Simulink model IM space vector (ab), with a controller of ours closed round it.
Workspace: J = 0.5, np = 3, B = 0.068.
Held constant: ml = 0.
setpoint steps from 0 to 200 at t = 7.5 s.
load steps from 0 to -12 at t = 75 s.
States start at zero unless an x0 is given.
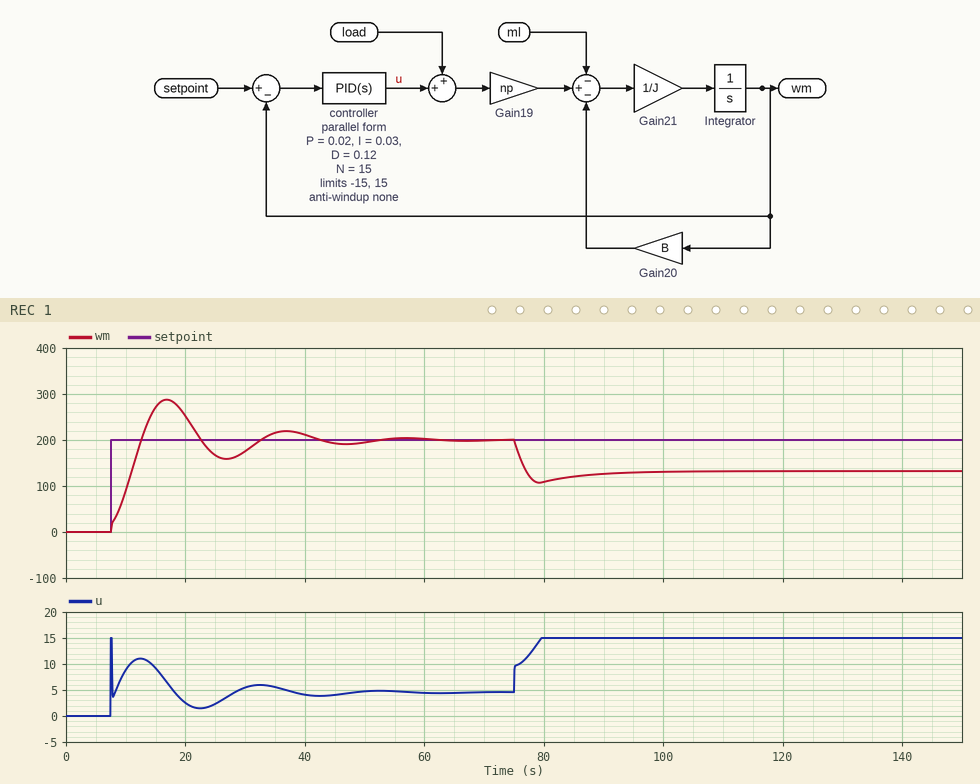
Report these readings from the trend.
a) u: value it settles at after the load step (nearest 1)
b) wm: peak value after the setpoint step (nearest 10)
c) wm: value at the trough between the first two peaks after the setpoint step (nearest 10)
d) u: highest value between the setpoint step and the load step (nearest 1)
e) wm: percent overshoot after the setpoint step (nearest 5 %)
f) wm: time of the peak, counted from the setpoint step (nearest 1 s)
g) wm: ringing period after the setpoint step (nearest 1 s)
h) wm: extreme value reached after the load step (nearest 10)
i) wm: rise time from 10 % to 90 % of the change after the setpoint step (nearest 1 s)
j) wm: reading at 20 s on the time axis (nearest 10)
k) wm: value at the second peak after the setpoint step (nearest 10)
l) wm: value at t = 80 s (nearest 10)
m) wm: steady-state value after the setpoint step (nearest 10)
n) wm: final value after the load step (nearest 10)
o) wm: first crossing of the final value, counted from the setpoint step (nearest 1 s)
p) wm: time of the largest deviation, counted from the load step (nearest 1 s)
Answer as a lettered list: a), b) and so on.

a) 15
b) 290
c) 160
d) 15
e) 45 %
f) 9 s
g) 20 s
h) 110
i) 4 s
j) 250
k) 220
l) 110
m) 200
n) 130
o) 5 s
p) 4 s
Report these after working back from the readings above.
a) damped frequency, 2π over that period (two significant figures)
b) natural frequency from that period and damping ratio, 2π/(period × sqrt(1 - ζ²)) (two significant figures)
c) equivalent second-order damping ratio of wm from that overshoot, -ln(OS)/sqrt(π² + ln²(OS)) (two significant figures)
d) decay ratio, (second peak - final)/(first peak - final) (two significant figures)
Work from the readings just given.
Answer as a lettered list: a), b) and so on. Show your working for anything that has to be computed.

a) 2π / 20 = 0.31 rad/s
b) 2π / (20 × sqrt(1 - 0.25²)) = 0.32 rad/s
c) ln(0.45) = -0.799; 0.799 / sqrt(9.870 + 0.638) = 0.25
d) (220 - 200) / (290 - 200) = 0.22
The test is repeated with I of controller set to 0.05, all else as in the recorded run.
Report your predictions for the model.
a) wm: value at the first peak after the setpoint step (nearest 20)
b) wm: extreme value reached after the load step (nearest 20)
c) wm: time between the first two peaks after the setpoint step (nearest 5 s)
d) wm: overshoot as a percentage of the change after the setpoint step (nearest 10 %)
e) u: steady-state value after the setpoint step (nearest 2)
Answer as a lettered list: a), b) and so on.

a) 300
b) 120
c) 15 s
d) 50 %
e) 4
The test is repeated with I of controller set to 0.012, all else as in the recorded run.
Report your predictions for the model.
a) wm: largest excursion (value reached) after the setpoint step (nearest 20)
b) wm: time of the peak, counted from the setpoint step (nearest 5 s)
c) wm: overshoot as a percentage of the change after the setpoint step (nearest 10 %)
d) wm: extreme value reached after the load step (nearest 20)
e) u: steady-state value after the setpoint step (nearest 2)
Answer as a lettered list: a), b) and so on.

a) 260
b) 15 s
c) 30 %
d) 80
e) 4
